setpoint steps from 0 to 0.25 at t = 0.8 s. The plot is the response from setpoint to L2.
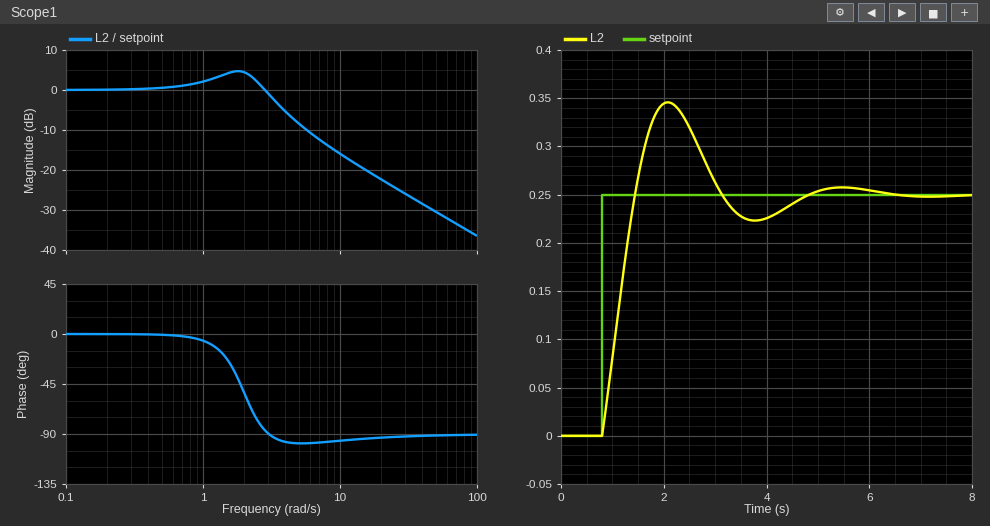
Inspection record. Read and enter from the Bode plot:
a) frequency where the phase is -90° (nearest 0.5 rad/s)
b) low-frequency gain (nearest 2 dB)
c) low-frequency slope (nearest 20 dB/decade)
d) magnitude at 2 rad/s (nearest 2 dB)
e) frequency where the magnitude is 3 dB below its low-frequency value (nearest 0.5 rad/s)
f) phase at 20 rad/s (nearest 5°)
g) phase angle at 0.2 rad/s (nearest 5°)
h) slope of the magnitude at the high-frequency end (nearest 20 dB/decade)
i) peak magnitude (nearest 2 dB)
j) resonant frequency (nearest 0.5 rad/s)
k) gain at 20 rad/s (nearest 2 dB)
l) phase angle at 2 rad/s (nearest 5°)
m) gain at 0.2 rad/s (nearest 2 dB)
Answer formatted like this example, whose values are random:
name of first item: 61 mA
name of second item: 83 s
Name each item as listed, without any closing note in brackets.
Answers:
frequency where the phase is -90°: 3.0 rad/s
low-frequency gain: 0 dB
low-frequency slope: 0 dB/decade
magnitude at 2 rad/s: 4 dB
frequency where the magnitude is 3 dB below its low-frequency value: 3.5 rad/s
phase at 20 rad/s: -95°
phase angle at 0.2 rad/s: 0°
slope of the magnitude at the high-frequency end: -20 dB/decade
peak magnitude: 4 dB
resonant frequency: 2.0 rad/s
gain at 20 rad/s: -22 dB
phase angle at 2 rad/s: -55°
gain at 0.2 rad/s: 0 dB
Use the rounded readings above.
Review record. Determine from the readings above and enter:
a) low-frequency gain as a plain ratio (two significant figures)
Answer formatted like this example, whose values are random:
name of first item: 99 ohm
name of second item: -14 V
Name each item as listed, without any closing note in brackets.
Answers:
low-frequency gain as a plain ratio: 1.0
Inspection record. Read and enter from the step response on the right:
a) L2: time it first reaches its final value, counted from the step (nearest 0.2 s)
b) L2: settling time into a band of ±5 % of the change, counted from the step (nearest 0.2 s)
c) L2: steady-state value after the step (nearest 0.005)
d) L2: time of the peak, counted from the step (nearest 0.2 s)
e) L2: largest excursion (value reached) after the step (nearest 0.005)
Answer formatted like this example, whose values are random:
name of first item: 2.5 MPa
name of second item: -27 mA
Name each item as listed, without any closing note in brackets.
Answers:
L2: time it first reaches its final value, counted from the step: 0.6 s
L2: settling time into a band of ±5 % of the change, counted from the step: 3.6 s
L2: steady-state value after the step: 0.250
L2: time of the peak, counted from the step: 1.2 s
L2: largest excursion (value reached) after the step: 0.345
